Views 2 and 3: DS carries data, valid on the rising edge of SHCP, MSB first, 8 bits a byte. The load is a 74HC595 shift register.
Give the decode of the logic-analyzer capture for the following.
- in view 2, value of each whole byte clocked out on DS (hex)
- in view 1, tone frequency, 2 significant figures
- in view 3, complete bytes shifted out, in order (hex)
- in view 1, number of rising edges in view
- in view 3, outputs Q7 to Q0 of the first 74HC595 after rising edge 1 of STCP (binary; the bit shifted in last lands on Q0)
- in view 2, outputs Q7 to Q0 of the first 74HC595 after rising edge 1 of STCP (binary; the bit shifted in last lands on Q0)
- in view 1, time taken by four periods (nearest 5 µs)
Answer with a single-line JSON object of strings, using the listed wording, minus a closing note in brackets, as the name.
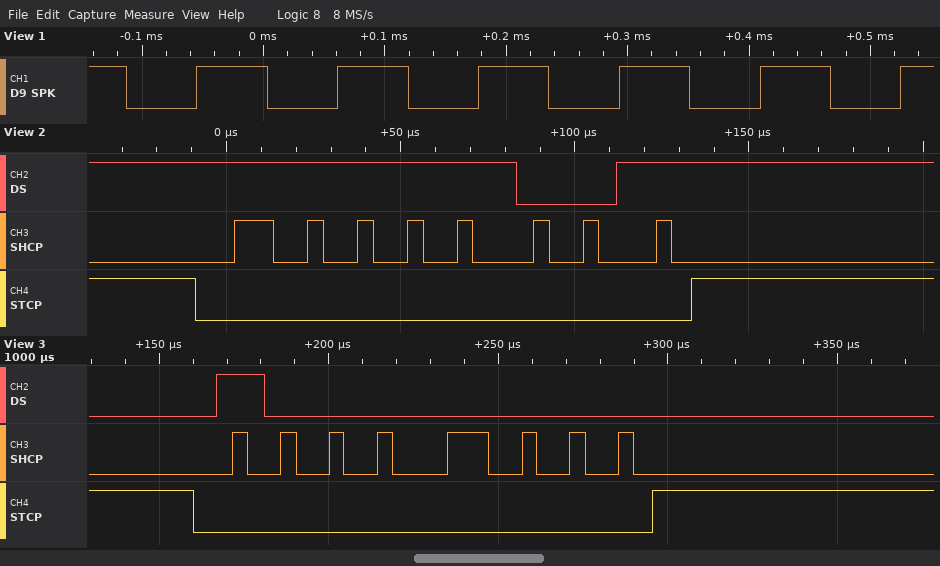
{"in view 2, value of each whole byte clocked out on DS": "0xF9", "in view 1, tone frequency, 2 significant figures": "8.6 kHz", "in view 3, complete bytes shifted out, in order": "0x80", "in view 1, number of rising edges in view": "6", "in view 3, outputs Q7 to Q0 of the first 74HC595 after rising edge 1 of STCP": "10000000", "in view 2, outputs Q7 to Q0 of the first 74HC595 after rising edge 1 of STCP": "11111001", "in view 1, time taken by four periods": "465 µs"}
